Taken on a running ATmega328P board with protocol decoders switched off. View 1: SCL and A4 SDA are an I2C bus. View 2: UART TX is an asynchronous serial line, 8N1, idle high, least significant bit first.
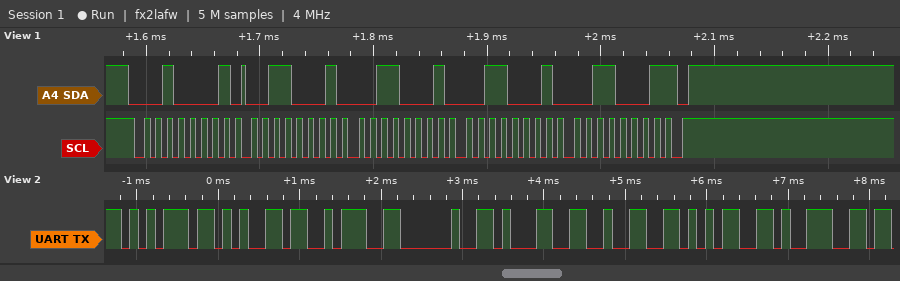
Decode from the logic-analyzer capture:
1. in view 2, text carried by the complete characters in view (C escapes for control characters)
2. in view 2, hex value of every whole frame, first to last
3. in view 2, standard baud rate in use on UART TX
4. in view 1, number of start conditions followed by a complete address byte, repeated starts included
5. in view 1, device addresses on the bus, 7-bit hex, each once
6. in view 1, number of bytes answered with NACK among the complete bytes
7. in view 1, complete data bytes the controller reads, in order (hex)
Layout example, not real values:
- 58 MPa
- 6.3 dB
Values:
- "ue: 1259"
- 75 65 3A 20 31 32 35 39
- 9600 baud
- 1
- 0x10
- 1
- 31 31 31 31
